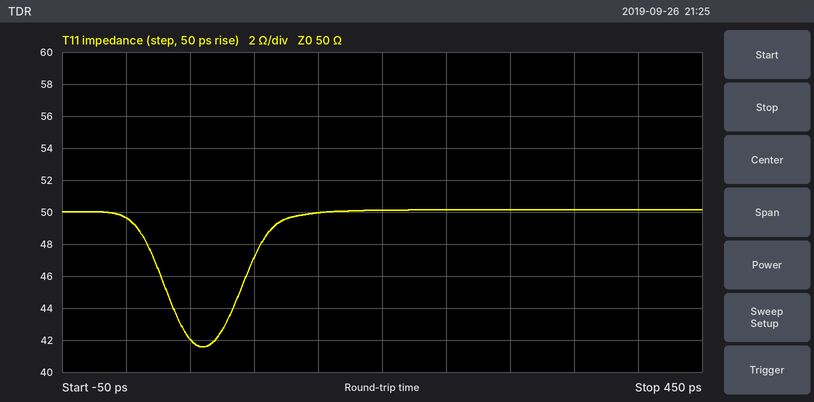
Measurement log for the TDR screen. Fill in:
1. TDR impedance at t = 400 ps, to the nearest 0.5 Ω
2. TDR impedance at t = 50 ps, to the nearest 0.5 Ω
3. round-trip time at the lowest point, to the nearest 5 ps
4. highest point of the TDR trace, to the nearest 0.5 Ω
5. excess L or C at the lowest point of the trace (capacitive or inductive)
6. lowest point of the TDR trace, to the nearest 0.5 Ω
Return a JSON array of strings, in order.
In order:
["50.0 Ω", "42.0 Ω", "60 ps", "50.0 Ω", "capacitive", "41.5 Ω"]
